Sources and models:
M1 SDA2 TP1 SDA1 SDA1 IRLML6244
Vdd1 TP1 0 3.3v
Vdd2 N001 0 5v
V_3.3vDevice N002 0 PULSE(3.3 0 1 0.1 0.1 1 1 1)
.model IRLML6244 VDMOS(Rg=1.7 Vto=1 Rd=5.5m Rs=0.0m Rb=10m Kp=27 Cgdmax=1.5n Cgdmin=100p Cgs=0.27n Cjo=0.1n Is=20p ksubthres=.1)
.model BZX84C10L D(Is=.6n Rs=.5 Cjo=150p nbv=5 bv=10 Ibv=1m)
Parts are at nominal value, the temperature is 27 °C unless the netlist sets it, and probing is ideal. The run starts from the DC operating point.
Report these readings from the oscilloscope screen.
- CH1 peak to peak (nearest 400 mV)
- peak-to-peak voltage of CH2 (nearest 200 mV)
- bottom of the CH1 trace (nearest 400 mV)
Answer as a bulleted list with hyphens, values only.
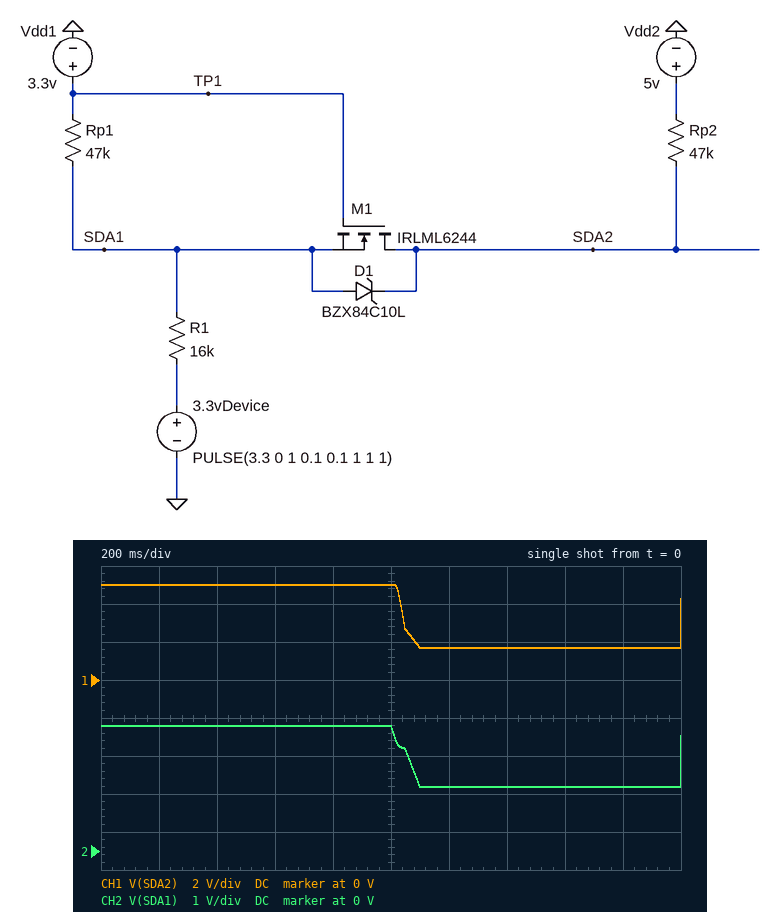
- 3.2 V
- 1.6 V
- 1.6 V
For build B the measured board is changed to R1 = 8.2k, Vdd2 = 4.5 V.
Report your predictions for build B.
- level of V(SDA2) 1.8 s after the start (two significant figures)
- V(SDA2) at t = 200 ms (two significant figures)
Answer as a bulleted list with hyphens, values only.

- 1.0 V
- 4.5 V
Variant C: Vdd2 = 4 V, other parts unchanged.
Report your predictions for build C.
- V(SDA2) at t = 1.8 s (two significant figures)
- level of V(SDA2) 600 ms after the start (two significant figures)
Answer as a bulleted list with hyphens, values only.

- 1.5 V
- 4.0 V
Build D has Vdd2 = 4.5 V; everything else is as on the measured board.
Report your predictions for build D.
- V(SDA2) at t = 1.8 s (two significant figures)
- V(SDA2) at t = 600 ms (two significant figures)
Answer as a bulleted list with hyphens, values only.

- 1.6 V
- 4.5 V
